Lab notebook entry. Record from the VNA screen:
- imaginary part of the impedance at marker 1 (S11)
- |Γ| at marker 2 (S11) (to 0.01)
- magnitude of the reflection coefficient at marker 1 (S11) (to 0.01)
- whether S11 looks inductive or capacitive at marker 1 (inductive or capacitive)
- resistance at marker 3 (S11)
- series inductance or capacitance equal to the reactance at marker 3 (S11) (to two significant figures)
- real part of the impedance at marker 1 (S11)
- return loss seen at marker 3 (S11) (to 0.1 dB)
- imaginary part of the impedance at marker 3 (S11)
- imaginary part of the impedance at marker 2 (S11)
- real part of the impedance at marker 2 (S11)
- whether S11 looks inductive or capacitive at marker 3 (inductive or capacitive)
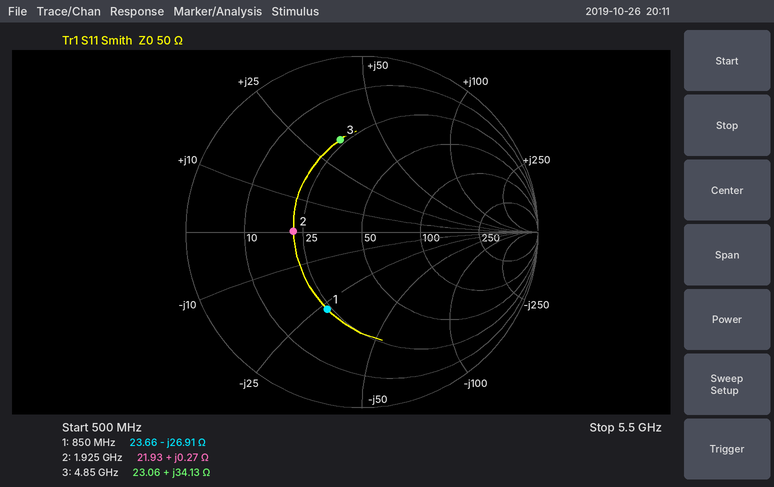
-26.91 Ω
0.39
0.48
capacitive
23.06 Ω
1.1 nH
23.66 Ω
5.4 dB
+34.13 Ω
+0.27 Ω
21.93 Ω
inductive
